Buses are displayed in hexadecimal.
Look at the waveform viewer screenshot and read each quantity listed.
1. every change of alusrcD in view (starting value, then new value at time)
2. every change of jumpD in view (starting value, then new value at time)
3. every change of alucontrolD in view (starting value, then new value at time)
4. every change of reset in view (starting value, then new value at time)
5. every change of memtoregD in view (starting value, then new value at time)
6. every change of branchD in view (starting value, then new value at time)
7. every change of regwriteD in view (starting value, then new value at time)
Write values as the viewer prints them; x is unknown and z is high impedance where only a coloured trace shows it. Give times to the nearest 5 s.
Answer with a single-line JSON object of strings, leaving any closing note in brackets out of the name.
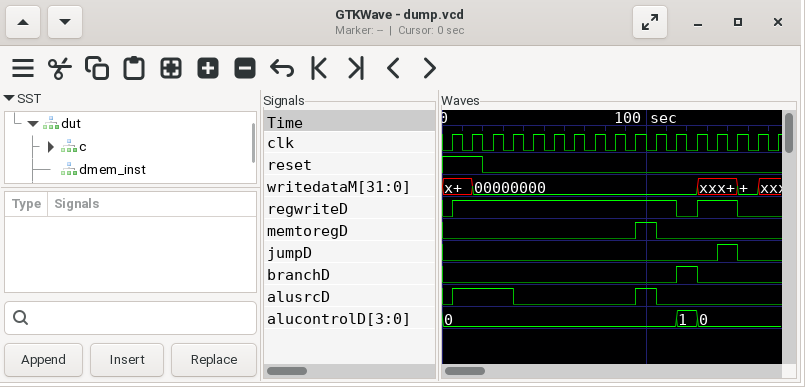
{"every change of alusrcD in view": "0, 1 at 5 s, 0 at 35 s, 1 at 95 s, 0 at 105 s", "every change of jumpD in view": "0, 1 at 135 s, 0 at 145 s", "every change of alucontrolD in view": "0, 1 at 115 s, 0 at 125 s", "every change of reset in view": "1, 0 at 20 s", "every change of memtoregD in view": "0, 1 at 95 s, 0 at 105 s", "every change of branchD in view": "0, 1 at 115 s, 0 at 125 s", "every change of regwriteD in view": "0, 1 at 5 s, 0 at 115 s, 1 at 125 s, 0 at 145 s"}
